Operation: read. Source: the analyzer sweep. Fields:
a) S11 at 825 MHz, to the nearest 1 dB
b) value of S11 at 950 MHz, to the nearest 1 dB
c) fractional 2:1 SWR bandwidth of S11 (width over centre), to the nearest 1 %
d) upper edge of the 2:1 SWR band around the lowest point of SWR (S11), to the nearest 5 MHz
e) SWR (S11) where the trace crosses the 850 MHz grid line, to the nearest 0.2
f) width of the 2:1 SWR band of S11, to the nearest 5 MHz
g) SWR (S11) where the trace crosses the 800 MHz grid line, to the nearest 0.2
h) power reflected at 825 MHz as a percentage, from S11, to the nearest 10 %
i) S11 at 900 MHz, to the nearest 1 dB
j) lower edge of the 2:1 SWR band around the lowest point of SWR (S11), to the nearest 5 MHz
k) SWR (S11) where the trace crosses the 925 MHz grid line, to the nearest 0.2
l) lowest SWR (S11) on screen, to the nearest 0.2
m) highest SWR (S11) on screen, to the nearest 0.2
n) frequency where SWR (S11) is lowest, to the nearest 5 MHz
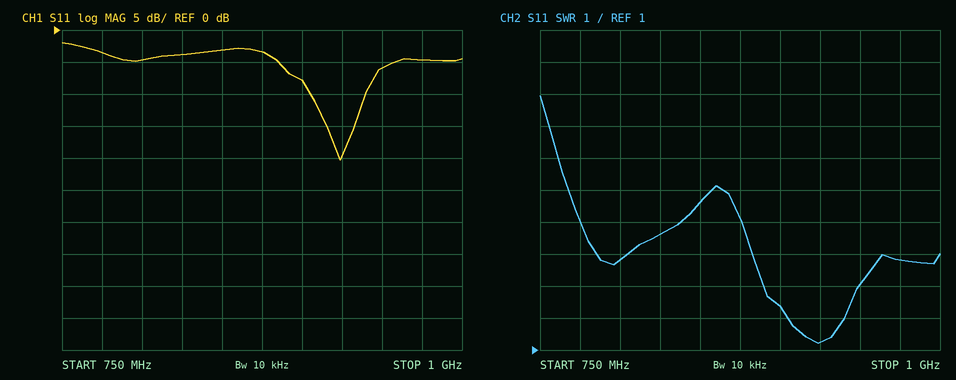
-4 dB
-6 dB
4 %
940 MHz
5.6
35 MHz
3.8
40 %
-8 dB
905 MHz
1.2
1.2
9.0
925 MHz
